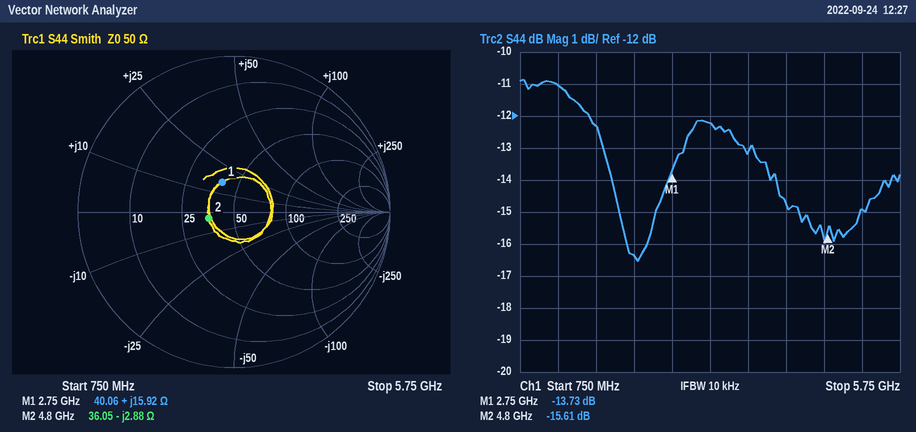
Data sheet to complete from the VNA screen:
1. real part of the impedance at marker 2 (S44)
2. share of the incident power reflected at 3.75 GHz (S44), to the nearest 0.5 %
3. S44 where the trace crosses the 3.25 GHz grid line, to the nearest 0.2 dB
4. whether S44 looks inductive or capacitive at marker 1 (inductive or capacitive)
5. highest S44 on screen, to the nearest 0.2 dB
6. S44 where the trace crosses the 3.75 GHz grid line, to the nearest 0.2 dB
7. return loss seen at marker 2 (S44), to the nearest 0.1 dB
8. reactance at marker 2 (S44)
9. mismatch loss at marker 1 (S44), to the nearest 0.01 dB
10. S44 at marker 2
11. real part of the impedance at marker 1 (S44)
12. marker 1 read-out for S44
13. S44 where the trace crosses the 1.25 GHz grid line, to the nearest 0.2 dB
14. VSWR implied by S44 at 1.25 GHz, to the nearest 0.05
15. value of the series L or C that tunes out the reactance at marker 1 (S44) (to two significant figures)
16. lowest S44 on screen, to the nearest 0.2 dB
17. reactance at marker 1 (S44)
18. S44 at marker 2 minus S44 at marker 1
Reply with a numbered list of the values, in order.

1. 36.05 Ω
2. 5.0 %
3. -12.2 dB
4. inductive
5. -10.8 dB
6. -13.2 dB
7. 15.6 dB
8. -2.88 Ω
9. 0.19 dB
10. -15.61 dB
11. 40.06 Ω
12. -13.73 dB
13. -11.0 dB
14. 1.80
15. 3.6 pF
16. -16.6 dB
17. +15.92 Ω
18. -1.88 dB
